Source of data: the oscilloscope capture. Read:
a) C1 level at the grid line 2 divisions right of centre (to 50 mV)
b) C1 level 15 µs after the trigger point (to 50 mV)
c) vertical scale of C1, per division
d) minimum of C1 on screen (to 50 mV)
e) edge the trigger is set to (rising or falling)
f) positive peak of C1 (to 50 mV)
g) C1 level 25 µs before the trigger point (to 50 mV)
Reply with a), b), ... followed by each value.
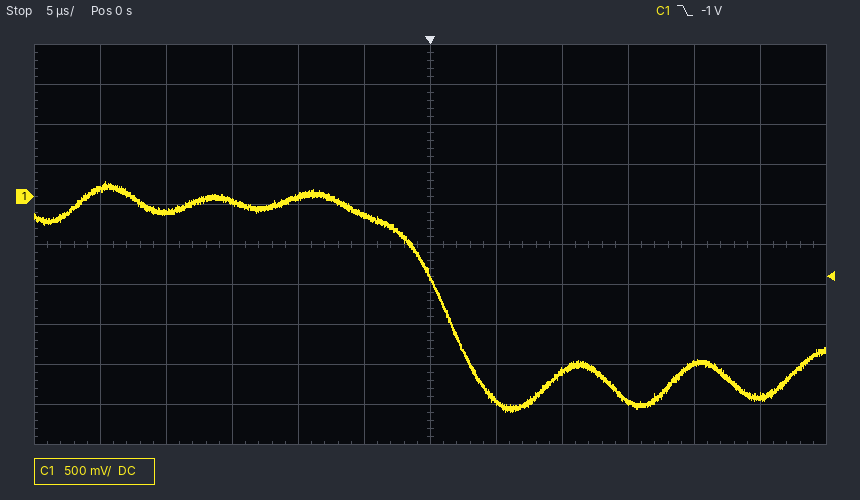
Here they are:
a) -2.20 V
b) -2.55 V
c) 500 mV
d) -2.70 V
e) falling
f) 200 mV
g) 100 mV
